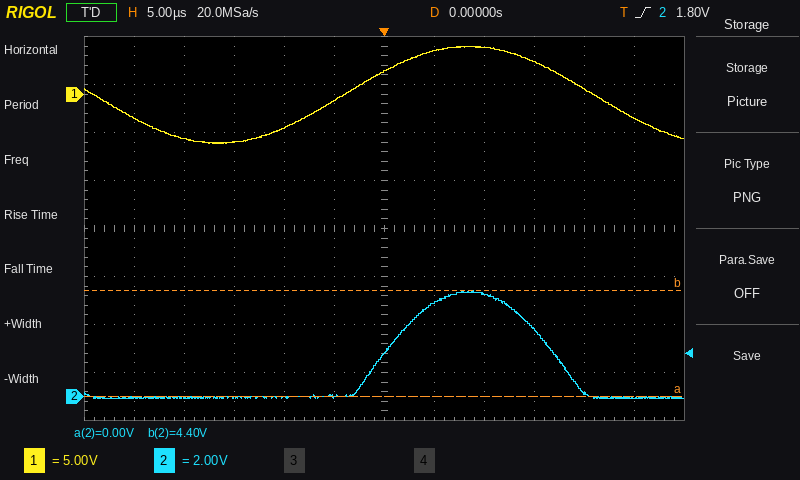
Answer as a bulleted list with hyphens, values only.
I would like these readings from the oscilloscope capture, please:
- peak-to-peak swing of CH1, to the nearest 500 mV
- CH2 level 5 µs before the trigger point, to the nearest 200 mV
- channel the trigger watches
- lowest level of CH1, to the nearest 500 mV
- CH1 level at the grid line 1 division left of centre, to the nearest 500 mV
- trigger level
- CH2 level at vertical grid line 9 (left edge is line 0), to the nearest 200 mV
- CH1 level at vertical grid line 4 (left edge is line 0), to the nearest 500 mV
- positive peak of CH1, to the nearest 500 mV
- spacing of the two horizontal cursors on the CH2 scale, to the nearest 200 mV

- 10.0 V
- 0.0 V
- CH2
- -5.0 V
- -500 mV
- 1.80 V
- 2.8 V
- -3.5 V
- 5.0 V
- 4.4 V
